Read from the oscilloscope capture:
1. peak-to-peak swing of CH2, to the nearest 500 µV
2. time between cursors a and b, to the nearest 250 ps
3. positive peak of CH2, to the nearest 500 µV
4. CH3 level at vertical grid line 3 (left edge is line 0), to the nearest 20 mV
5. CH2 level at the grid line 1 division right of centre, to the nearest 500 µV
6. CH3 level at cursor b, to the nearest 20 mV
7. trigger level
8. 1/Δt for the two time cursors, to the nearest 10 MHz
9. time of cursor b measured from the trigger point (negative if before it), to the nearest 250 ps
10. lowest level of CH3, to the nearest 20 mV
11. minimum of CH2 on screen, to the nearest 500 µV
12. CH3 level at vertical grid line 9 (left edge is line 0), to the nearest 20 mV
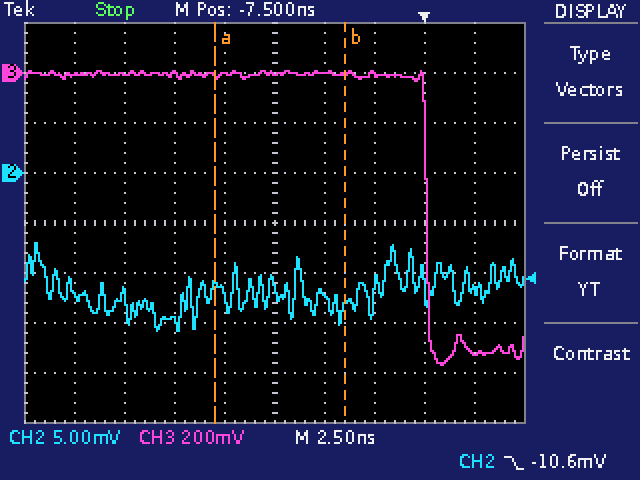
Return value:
9.0 mV
6.50 ns
-7.0 mV
0 mV
-12.0 mV
0 mV
-10.6 mV
150 MHz
-4.00 ns
-1.16 V
-16.0 mV
-1.12 V
